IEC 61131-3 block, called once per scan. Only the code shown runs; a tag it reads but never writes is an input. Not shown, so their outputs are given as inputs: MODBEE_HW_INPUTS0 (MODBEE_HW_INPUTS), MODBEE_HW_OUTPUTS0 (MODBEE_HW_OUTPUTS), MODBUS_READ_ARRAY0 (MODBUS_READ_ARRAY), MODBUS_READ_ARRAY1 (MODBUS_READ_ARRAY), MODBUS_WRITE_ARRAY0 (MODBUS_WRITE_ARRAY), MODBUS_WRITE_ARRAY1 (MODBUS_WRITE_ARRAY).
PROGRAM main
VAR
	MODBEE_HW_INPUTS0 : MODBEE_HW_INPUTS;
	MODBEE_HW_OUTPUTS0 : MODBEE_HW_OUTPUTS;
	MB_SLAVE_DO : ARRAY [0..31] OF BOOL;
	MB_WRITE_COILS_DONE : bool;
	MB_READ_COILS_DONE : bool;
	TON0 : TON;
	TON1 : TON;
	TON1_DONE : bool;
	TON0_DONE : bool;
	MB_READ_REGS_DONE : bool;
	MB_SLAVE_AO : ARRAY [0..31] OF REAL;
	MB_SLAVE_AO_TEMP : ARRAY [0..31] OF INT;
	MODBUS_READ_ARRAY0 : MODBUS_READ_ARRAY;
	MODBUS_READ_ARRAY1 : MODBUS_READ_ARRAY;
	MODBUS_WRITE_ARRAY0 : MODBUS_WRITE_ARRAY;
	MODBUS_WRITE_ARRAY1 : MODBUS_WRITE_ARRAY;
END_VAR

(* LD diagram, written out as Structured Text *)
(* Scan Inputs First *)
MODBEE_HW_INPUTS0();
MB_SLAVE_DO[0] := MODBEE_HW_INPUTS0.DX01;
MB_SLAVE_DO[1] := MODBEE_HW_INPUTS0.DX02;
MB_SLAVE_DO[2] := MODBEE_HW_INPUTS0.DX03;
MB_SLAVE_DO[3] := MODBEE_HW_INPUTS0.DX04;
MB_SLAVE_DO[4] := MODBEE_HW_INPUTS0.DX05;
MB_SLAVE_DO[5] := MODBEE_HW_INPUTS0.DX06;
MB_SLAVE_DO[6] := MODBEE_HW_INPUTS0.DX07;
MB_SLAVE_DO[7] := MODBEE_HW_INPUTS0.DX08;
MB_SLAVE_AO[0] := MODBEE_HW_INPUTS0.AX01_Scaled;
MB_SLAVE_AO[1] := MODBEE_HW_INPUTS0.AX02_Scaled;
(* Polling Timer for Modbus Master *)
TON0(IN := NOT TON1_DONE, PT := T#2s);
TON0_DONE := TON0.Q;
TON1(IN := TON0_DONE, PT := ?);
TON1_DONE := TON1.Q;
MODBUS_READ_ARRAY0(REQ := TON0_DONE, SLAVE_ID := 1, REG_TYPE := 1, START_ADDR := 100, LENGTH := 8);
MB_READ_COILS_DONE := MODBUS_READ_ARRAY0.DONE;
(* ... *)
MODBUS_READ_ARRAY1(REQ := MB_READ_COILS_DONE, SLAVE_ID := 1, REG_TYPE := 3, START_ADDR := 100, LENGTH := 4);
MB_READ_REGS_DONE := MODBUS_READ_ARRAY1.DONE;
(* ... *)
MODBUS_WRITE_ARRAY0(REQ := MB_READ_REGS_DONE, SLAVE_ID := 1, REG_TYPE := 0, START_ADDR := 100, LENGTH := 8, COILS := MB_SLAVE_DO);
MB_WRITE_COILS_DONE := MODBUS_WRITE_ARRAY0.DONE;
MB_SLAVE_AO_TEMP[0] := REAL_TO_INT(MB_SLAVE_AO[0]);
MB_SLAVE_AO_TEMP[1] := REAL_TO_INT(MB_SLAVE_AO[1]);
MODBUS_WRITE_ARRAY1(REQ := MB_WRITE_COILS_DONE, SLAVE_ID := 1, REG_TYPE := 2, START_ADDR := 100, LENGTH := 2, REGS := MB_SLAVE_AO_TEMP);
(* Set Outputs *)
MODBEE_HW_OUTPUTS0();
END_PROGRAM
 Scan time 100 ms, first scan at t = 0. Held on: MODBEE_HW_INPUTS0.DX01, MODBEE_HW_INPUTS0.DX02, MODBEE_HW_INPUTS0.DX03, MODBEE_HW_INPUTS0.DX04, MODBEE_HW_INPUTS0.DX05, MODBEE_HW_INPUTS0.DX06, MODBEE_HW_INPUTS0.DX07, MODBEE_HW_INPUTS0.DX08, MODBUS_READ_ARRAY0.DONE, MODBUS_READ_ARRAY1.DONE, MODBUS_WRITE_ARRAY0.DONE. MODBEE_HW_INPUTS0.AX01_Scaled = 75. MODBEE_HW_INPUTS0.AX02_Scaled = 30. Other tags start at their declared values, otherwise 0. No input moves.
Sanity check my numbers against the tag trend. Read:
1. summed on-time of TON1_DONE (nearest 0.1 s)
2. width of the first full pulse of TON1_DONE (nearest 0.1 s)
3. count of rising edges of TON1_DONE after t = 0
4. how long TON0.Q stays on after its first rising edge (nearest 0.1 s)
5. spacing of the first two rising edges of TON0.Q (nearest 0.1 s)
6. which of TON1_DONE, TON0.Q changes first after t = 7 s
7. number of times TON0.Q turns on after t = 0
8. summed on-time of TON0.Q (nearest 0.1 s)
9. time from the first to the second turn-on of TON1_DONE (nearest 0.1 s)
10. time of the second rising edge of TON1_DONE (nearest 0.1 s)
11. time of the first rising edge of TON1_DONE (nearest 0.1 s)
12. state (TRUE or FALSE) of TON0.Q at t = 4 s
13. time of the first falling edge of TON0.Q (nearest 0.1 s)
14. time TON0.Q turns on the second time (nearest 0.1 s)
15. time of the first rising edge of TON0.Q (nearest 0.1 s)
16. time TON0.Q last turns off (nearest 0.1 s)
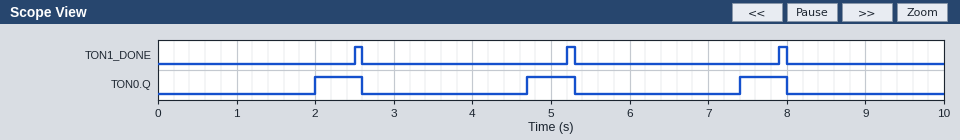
0.3 s
0.1 s
3
0.6 s
2.7 s
TON0.Q
3
1.8 s
2.7 s
5.2 s
2.5 s
FALSE
2.6 s
4.7 s
2.0 s
8.0 s
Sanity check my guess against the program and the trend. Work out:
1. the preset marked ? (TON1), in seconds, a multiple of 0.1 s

0.5 s
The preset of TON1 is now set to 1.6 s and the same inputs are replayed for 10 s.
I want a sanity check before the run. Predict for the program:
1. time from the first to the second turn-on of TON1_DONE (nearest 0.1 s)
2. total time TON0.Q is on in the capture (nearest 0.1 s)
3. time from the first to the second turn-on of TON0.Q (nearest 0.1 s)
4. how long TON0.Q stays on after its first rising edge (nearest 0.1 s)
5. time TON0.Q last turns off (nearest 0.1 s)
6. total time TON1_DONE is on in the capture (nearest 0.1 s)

3.8 s
3.8 s
3.8 s
1.7 s
7.5 s
0.2 s
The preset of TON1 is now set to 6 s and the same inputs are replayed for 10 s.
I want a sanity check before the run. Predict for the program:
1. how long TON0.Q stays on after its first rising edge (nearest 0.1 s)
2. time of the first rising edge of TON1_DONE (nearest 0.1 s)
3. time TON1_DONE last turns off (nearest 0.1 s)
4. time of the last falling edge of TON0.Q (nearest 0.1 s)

6.1 s
8.0 s
8.1 s
8.1 s
